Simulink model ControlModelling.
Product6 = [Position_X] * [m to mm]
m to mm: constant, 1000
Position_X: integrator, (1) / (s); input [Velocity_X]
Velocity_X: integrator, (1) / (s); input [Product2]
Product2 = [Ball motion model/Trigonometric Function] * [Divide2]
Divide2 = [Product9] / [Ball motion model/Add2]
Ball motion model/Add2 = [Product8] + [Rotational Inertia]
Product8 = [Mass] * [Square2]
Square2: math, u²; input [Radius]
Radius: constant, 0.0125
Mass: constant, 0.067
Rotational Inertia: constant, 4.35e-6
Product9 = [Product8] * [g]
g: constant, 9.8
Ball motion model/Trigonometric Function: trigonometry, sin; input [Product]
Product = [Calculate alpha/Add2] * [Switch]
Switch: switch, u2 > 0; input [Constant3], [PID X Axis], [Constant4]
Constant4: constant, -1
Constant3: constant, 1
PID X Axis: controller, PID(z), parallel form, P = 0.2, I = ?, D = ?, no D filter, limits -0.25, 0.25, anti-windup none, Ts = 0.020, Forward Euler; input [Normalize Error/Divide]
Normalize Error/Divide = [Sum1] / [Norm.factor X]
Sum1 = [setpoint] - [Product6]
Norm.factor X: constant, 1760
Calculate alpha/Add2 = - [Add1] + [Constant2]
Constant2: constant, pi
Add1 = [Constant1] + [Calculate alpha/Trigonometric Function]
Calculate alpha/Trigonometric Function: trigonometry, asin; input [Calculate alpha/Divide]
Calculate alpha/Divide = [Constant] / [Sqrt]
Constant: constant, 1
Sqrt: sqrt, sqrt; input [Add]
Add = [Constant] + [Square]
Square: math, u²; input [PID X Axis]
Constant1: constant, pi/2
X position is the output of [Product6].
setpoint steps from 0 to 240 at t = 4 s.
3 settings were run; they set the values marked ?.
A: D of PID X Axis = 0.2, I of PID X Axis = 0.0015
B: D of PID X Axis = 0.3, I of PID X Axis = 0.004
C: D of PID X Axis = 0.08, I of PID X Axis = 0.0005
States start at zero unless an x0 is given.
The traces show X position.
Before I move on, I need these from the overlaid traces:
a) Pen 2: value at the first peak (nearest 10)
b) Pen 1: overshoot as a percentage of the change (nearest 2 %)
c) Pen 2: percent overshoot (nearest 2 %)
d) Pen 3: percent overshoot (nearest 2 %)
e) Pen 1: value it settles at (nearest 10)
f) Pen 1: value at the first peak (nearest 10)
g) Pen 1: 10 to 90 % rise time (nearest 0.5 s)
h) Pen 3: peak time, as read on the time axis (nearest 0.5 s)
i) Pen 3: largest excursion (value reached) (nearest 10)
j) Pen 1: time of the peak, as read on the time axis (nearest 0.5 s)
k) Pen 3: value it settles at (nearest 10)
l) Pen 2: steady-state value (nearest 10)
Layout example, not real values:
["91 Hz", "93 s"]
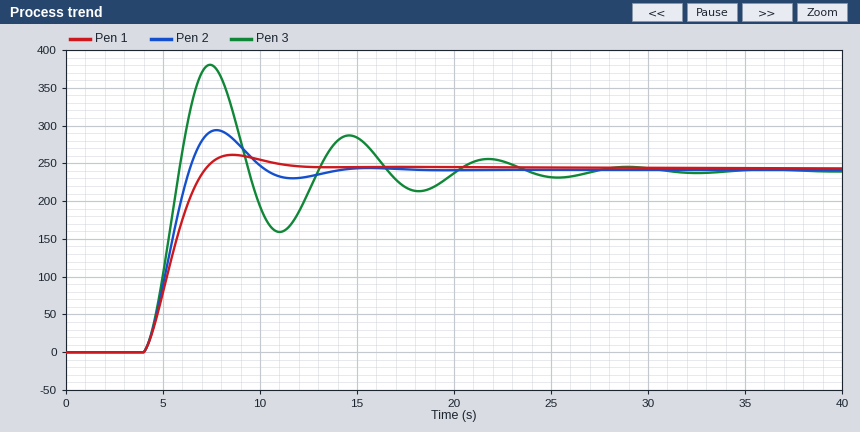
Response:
["290", "8 %", "22 %", "58 %", "240", "260", "2.0 s", "7.5 s", "380", "8.5 s", "240", "240"]
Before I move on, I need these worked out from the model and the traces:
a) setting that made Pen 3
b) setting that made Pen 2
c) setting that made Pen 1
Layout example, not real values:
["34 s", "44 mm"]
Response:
["C", "A", "B"]
